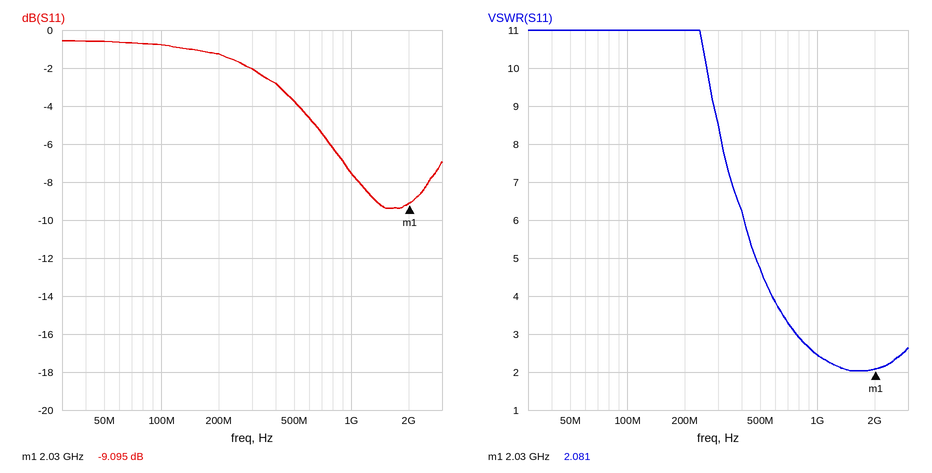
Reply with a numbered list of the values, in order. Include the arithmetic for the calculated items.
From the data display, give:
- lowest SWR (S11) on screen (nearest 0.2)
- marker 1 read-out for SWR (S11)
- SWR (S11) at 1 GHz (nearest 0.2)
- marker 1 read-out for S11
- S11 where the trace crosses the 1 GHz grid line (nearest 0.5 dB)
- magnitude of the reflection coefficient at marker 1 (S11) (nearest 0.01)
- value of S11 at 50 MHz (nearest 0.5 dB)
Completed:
1. 2.0
2. 2.081
3. 2.4
4. -9.095 dB
5. -7.5 dB
6. 10^(-9.095/20) ≈ 0.35
7. -0.5 dB
